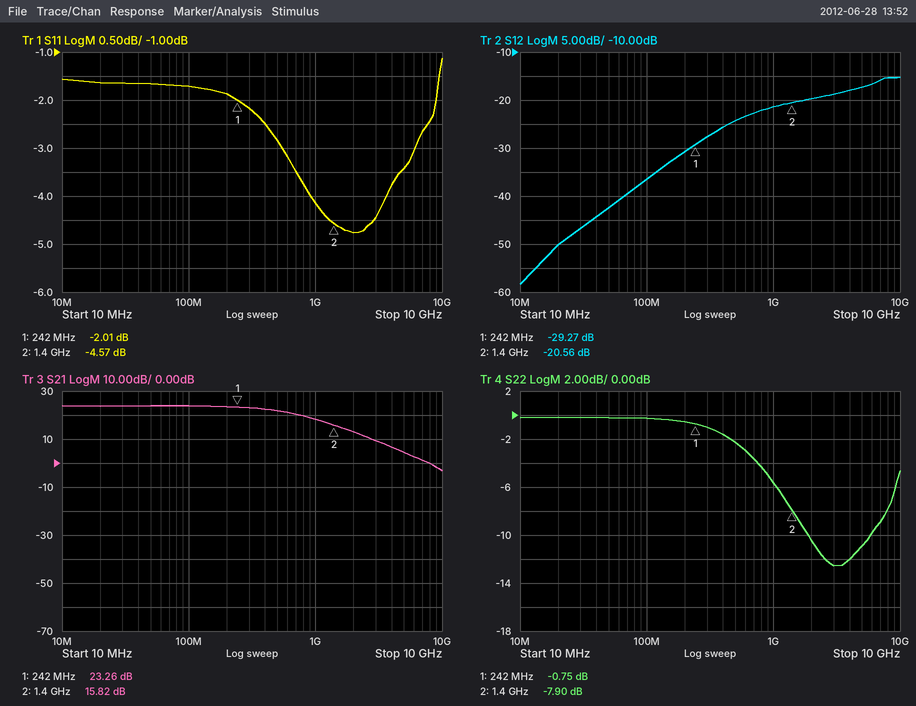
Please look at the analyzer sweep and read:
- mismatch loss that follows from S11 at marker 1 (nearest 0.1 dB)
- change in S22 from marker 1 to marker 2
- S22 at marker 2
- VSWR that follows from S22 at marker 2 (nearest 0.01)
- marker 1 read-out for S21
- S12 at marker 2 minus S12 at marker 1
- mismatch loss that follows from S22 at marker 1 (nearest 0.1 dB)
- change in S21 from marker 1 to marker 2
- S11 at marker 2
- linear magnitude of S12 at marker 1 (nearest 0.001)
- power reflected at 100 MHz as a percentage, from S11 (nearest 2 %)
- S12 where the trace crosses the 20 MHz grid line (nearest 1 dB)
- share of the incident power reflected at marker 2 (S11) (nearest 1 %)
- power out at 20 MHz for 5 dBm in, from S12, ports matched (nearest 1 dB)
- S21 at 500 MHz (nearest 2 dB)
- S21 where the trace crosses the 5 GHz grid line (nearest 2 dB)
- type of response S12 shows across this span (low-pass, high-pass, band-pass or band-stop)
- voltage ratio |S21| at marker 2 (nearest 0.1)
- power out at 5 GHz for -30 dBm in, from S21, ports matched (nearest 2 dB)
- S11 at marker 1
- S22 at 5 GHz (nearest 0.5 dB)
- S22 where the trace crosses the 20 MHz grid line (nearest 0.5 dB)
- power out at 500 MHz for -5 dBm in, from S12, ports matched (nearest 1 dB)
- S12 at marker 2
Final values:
4.3 dB
-7.15 dB
-7.90 dB
2.35
23.26 dB
8.71 dB
8.0 dB
-7.44 dB
-4.57 dB
0.034
68 %
-50 dB
35 %
-45 dBm
22 dB
4 dB
high-pass
6.2
-26 dBm
-2.01 dB
-11.0 dB
0.0 dB
-29 dBm
-20.56 dB
